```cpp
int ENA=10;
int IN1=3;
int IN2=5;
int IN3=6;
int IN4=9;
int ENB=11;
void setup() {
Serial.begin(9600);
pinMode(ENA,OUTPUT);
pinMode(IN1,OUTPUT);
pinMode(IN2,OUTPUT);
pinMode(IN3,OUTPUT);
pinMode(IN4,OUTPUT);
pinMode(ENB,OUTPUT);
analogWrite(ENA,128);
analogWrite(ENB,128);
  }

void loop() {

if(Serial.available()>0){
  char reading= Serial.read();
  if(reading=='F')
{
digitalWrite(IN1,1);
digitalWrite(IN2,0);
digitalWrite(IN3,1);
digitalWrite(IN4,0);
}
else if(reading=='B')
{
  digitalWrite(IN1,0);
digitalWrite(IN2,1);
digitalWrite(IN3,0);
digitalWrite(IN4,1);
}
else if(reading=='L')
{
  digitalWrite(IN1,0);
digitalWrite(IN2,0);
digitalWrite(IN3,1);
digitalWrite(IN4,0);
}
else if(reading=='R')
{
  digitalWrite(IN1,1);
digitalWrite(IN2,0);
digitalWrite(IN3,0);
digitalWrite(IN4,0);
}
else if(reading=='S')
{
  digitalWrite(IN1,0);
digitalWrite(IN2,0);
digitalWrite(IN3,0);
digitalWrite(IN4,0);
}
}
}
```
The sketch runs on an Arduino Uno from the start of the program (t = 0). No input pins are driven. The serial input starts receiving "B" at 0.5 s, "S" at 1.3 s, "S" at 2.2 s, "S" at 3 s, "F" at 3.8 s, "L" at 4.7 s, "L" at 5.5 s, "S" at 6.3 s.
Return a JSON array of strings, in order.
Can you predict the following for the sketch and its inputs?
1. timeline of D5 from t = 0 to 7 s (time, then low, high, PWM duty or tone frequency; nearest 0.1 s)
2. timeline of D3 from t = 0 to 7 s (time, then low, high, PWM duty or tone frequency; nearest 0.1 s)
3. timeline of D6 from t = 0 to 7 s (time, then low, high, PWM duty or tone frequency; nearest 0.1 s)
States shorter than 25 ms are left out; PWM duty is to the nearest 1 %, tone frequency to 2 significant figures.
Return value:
["0 s low; 0.5 s high; 1.3 s low", "0 s low; 3.8 s high; 4.7 s low", "0 s low; 3.8 s high; 6.3 s low"]
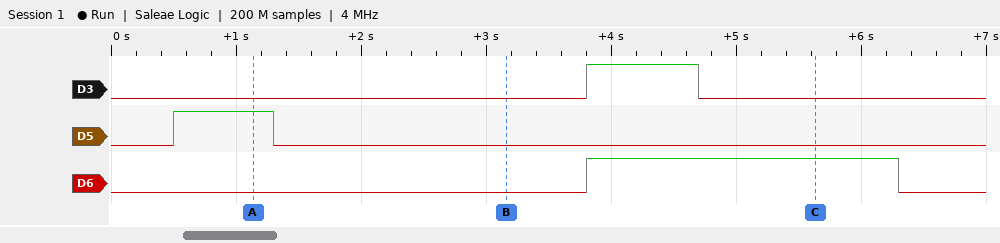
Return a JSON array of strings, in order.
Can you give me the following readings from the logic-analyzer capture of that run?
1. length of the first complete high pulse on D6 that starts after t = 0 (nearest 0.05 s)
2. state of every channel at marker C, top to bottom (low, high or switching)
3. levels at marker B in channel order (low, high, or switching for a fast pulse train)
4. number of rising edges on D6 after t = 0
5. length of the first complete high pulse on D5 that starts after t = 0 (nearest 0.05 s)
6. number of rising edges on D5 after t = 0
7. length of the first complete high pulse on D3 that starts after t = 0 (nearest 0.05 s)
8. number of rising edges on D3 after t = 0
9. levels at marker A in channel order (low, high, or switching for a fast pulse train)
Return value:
["2.50 s", "D3 low, D5 low, D6 high", "D3 low, D5 low, D6 low", "1", "0.80 s", "1", "0.90 s", "1", "D3 low, D5 high, D6 low"]
